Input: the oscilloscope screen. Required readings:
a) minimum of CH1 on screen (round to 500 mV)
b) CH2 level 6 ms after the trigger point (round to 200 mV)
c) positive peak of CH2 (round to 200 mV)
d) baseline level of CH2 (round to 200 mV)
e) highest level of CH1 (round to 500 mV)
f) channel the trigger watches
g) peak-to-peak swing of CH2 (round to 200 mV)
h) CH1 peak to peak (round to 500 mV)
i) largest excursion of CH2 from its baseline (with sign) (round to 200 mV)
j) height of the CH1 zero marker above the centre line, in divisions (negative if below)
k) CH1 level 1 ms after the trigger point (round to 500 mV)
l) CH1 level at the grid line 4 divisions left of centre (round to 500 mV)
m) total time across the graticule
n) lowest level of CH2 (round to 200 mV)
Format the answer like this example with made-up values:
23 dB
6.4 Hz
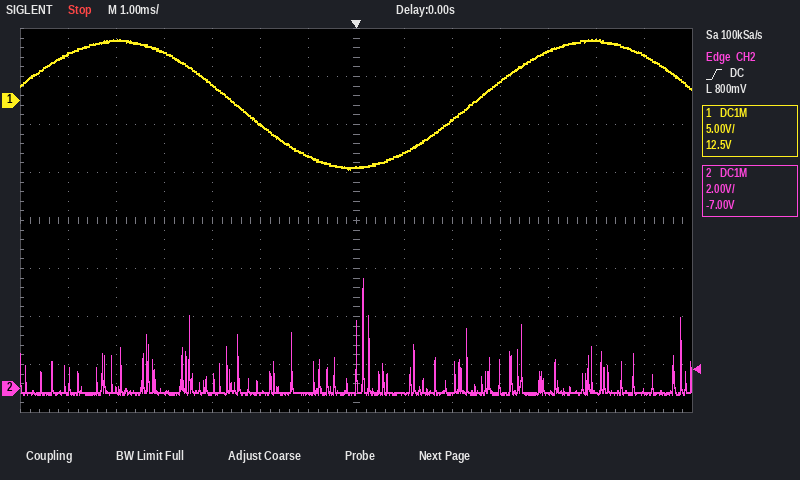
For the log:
-7.0 V
-200 mV
4.6 V
-200 mV
6.5 V
CH2
4.8 V
13.5 V
+4.8 V
+2.5 div
-5.5 V
5.0 V
14 ms
-200 mV
